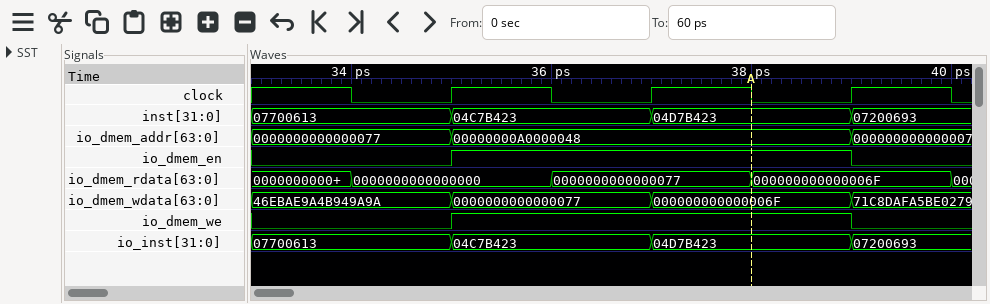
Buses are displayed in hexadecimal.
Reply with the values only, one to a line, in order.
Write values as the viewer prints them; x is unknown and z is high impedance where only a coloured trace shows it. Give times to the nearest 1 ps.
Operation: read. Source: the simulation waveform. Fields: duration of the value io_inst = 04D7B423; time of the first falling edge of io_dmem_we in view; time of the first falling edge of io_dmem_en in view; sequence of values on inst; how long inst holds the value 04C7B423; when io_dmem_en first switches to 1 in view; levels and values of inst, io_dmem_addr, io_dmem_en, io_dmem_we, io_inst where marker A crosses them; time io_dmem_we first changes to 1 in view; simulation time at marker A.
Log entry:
2 ps
39 ps
39 ps
07700613, 04C7B423, 04D7B423, 07200693
2 ps
35 ps
inst=04D7B423, io_dmem_addr=00000000A0000048, io_dmem_en=1, io_dmem_we=1, io_inst=04D7B423
35 ps
38 ps
